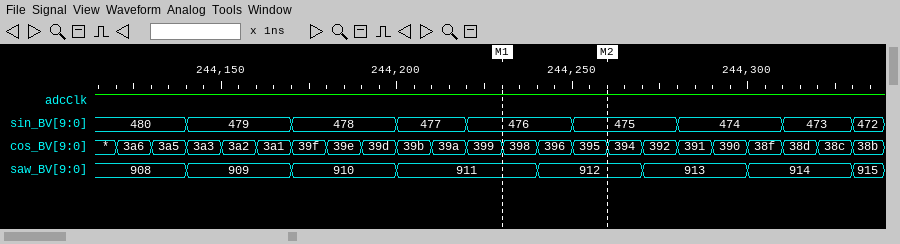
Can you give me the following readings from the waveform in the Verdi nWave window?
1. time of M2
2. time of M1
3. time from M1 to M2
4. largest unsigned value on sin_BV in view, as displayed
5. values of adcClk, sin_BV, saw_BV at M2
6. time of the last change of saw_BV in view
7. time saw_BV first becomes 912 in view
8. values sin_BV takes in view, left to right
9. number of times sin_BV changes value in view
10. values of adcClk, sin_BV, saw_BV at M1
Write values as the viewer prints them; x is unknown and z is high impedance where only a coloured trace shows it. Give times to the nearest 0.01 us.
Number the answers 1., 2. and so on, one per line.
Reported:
1. 244.26 us
2. 244.23 us
3. 0.03 us
4. 480
5. adcClk=1, sin_BV=475, saw_BV=912
6. 244.33 us
7. 244.24 us
8. 480, 479, 478, 477, 476, 475, 474, 473, 472
9. 8
10. adcClk=1, sin_BV=476, saw_BV=911
